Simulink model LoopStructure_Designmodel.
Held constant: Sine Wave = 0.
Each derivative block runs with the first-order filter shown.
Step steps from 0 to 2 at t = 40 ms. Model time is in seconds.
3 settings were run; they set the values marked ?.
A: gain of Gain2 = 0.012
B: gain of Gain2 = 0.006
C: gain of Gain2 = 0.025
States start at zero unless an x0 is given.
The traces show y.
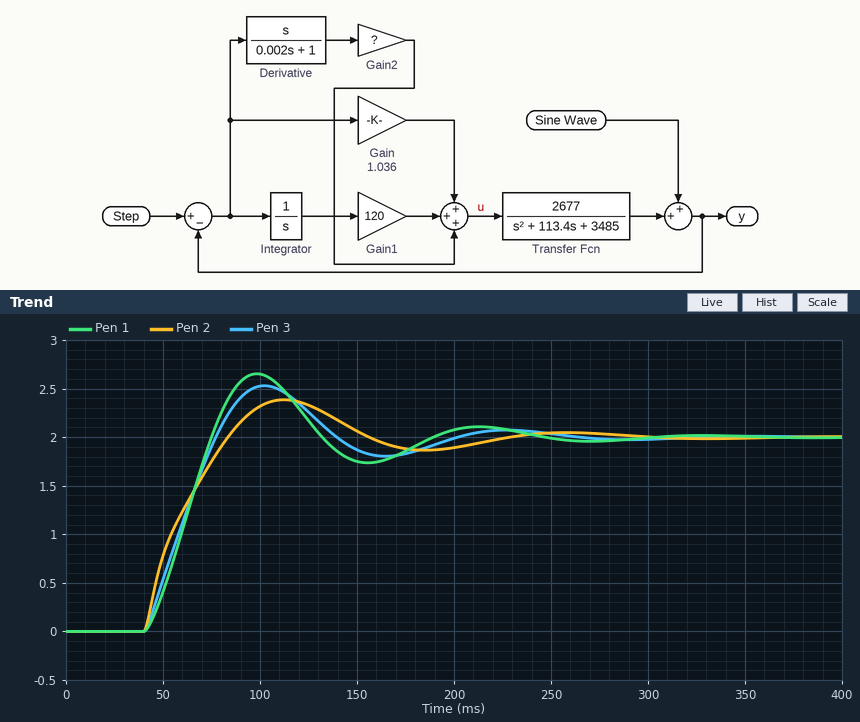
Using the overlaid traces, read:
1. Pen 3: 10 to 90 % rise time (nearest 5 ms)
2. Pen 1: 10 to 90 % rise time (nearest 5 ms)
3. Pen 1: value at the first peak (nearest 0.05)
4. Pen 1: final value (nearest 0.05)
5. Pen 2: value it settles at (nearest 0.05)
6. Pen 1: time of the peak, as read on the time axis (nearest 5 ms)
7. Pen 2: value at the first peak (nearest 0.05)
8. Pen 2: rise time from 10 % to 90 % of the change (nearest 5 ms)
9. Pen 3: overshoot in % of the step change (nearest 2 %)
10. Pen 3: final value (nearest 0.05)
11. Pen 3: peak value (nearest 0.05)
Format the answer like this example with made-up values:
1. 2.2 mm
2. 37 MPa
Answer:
1. 30 ms
2. 25 ms
3. 2.65
4. 2.00
5. 2.00
6. 100 ms
7. 2.40
8. 35 ms
9. 26 %
10. 2.00
11. 2.55
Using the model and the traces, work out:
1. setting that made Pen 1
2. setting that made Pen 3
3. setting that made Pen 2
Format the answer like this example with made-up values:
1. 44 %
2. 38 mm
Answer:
1. B
2. A
3. C
